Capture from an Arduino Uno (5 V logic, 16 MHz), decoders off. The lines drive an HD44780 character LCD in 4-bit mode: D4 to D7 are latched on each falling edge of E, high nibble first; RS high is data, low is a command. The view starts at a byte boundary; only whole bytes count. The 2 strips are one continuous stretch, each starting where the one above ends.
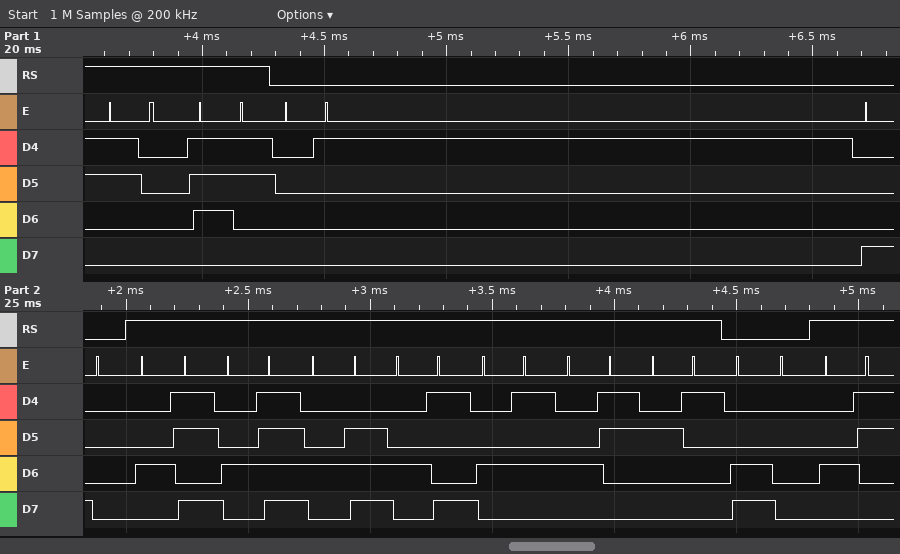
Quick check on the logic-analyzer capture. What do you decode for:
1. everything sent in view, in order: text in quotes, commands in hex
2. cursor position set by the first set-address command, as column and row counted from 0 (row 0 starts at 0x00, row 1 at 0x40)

"0s" 0x01 0x80 "KONIEC!" 0xC0 "C"
column 0, row 0
